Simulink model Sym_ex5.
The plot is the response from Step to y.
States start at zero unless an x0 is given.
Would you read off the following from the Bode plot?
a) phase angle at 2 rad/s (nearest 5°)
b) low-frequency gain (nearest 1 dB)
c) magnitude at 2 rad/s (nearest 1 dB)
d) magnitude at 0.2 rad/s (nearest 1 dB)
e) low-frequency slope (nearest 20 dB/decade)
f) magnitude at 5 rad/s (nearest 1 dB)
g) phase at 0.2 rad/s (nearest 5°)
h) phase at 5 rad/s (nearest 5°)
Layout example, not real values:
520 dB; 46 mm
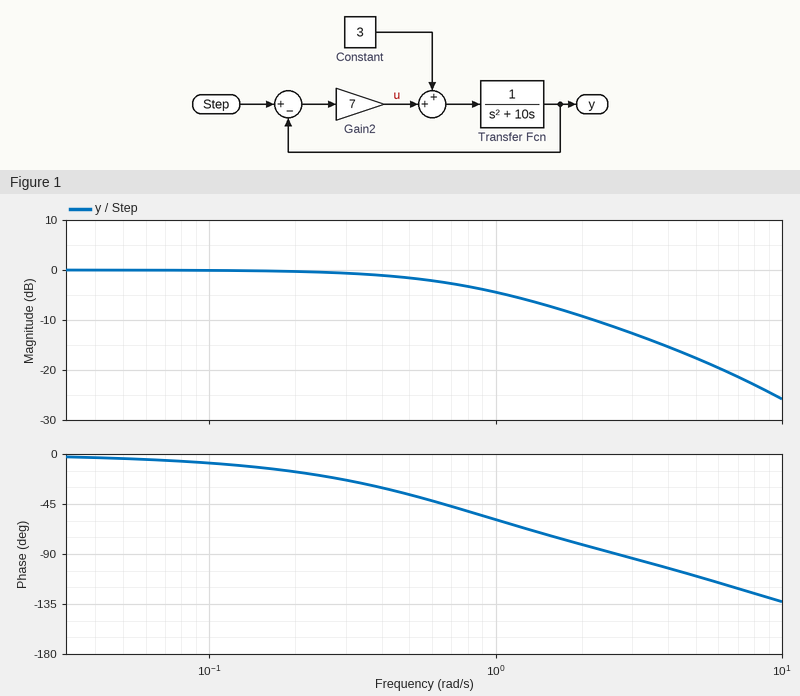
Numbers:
-80°; 0 dB; -9 dB; 0 dB; 0 dB/decade; -18 dB; -15°; -110°
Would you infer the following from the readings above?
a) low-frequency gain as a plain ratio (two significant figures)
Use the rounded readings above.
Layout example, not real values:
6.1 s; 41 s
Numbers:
1.0
